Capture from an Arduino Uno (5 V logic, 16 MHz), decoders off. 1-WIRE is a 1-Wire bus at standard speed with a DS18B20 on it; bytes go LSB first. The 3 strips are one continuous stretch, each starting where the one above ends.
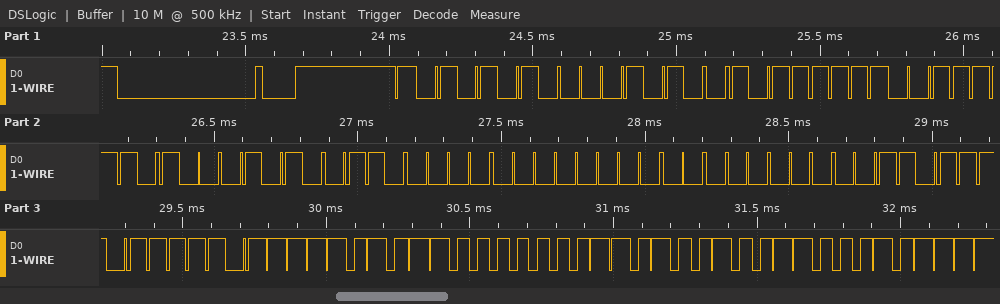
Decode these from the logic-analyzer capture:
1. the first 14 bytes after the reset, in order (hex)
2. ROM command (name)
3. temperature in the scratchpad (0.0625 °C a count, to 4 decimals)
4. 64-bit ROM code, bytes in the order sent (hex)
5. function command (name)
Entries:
55 28 FD 7C 51 06 00 00 EC BE AF 01 4B 46
Match ROM
26.9375 °C
28 FD 7C 51 06 00 00 EC
Read Scratchpad
